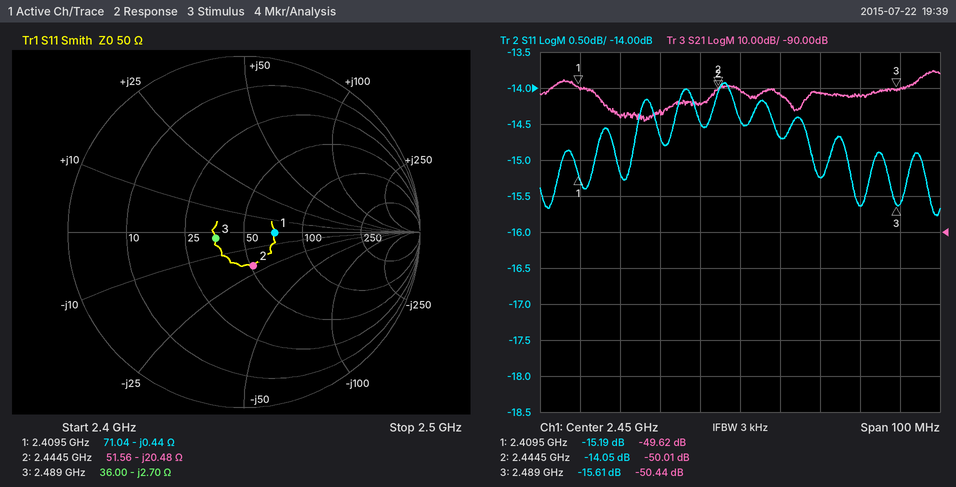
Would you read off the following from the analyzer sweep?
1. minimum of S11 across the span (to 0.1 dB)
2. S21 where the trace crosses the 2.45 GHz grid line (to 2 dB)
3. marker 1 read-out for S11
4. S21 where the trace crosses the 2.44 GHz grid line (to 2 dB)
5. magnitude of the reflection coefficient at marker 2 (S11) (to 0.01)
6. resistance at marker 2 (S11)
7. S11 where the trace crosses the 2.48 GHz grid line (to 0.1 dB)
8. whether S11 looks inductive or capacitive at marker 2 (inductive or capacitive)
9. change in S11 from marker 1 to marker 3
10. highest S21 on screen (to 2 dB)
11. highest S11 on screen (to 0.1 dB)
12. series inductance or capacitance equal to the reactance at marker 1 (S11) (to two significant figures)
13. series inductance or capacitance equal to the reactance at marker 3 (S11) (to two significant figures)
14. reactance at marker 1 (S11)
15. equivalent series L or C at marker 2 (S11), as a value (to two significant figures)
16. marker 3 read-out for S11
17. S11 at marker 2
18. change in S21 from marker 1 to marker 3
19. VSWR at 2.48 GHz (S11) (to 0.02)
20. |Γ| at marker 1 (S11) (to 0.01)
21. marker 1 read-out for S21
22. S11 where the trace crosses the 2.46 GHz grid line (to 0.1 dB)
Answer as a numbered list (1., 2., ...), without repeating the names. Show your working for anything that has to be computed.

1. -15.8 dB
2. -50 dB
3. -15.19 dB
4. -54 dB
5. 0.20
6. 51.56 Ω
7. -15.6 dB
8. capacitive
9. -15.61 − (-15.19) = -0.42 dB
10. -46 dB
11. -13.9 dB
12. C = 1/(2π × 2.4095 GHz × 0.44 Ω) ≈ 150 pF
13. C = 1/(2π × 2.489 GHz × 2.7 Ω) ≈ 24 pF
14. -0.44 Ω
15. C = 1/(2π × 2.4445 GHz × 20.48 Ω) ≈ 3.2 pF
16. -15.61 dB
17. -14.05 dB
18. -50.44 − (-49.62) = -0.82 dB
19. |Γ| = 10^(-15.6/20) = 0.1660; VSWR = (1 + 0.1660)/(1 − 0.1660) ≈ 1.40
20. 0.17
21. -49.62 dB
22. -14.7 dB
